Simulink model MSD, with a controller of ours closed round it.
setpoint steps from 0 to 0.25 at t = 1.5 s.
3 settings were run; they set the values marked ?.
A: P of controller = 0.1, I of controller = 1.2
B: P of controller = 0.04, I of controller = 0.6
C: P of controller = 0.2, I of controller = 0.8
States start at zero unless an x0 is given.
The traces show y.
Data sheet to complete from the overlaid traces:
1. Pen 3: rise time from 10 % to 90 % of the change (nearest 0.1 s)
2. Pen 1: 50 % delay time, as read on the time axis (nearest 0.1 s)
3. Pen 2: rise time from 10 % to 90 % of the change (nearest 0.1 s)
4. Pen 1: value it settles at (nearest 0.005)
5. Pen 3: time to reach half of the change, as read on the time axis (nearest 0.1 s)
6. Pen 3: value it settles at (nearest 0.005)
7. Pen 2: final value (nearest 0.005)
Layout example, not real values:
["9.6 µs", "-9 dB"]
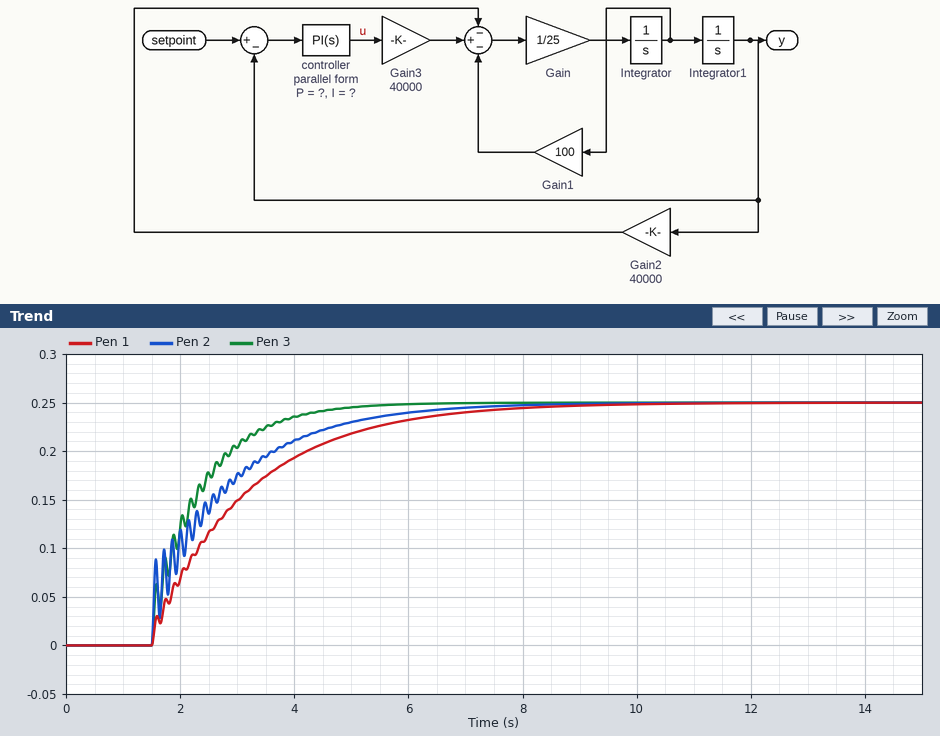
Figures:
["2.0 s", "2.6 s", "3.2 s", "0.250", "2.0 s", "0.250", "0.250"]
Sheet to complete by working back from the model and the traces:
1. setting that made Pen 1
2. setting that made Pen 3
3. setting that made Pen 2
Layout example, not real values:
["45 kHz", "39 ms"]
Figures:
["B", "A", "C"]
